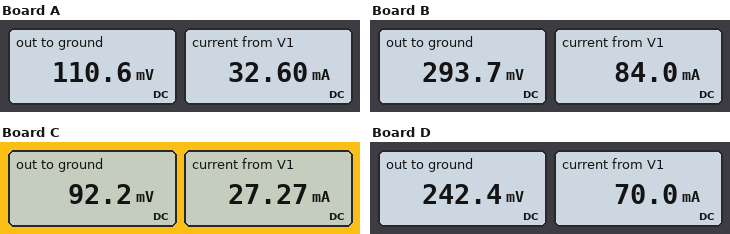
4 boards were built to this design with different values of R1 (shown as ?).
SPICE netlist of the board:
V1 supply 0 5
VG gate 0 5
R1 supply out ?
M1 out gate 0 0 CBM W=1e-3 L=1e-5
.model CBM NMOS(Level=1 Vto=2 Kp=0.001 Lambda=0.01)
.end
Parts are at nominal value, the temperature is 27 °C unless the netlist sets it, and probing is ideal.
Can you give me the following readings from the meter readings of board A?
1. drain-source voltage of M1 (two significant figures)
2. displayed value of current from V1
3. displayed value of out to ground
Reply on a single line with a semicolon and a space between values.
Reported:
110 mV; 32.60 mA; 110.6 mV
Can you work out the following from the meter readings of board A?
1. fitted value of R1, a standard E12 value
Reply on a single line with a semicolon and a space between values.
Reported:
150 Ω
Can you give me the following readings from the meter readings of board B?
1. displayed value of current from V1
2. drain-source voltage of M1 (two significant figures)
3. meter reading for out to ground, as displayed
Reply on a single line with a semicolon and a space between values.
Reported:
84.0 mA; 290 mV; 293.7 mV
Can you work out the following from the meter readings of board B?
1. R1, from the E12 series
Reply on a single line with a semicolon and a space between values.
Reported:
56 Ω
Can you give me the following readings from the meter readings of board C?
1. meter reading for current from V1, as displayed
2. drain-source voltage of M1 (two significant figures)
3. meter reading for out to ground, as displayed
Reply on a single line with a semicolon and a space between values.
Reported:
27.27 mA; 92 mV; 92.2 mV
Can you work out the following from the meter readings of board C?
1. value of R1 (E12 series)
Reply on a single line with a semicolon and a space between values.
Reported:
180 Ω
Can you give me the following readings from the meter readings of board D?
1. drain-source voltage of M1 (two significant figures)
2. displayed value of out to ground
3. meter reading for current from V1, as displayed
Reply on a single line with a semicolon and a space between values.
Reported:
240 mV; 242.4 mV; 70.0 mA
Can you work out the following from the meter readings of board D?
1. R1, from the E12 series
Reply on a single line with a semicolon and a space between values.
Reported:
68 Ω
